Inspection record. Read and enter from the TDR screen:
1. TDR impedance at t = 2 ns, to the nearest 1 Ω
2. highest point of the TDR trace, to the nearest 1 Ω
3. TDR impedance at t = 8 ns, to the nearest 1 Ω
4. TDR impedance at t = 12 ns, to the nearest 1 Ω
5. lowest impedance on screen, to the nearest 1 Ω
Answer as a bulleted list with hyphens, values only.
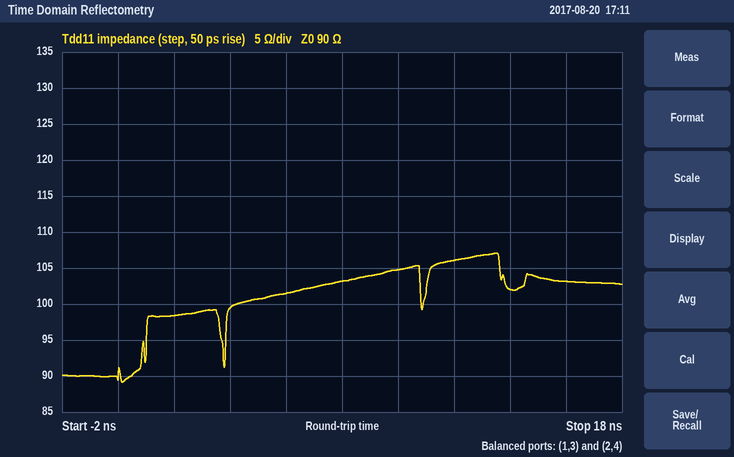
- 98 Ω
- 107 Ω
- 103 Ω
- 106 Ω
- 89 Ω
